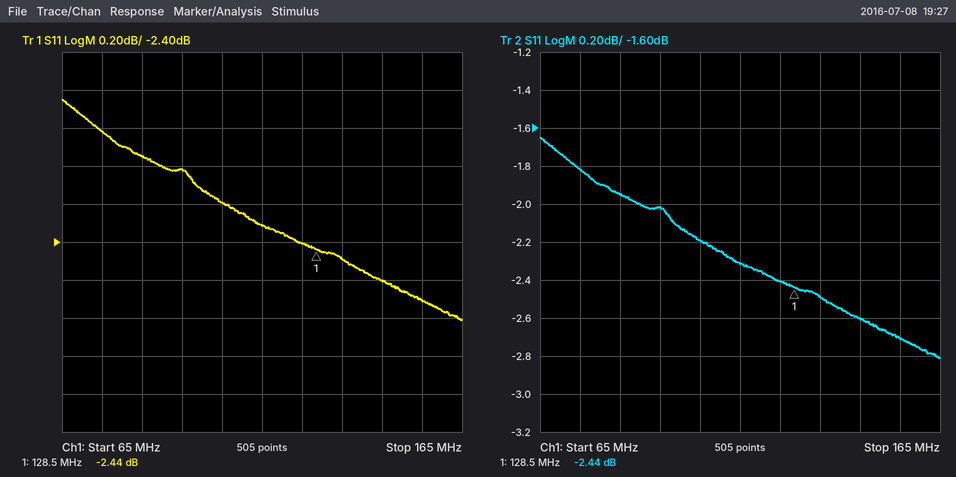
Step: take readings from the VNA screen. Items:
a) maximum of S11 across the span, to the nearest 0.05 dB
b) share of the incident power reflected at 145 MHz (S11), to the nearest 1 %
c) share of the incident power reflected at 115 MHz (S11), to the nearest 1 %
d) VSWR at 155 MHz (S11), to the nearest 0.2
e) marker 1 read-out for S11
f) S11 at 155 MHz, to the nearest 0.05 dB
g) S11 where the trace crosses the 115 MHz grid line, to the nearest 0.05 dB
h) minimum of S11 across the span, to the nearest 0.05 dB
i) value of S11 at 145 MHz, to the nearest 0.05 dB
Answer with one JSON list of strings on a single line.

["-1.65 dB", "55 %", "59 %", "6.4", "-2.44 dB", "-2.70 dB", "-2.30 dB", "-2.80 dB", "-2.60 dB"]
